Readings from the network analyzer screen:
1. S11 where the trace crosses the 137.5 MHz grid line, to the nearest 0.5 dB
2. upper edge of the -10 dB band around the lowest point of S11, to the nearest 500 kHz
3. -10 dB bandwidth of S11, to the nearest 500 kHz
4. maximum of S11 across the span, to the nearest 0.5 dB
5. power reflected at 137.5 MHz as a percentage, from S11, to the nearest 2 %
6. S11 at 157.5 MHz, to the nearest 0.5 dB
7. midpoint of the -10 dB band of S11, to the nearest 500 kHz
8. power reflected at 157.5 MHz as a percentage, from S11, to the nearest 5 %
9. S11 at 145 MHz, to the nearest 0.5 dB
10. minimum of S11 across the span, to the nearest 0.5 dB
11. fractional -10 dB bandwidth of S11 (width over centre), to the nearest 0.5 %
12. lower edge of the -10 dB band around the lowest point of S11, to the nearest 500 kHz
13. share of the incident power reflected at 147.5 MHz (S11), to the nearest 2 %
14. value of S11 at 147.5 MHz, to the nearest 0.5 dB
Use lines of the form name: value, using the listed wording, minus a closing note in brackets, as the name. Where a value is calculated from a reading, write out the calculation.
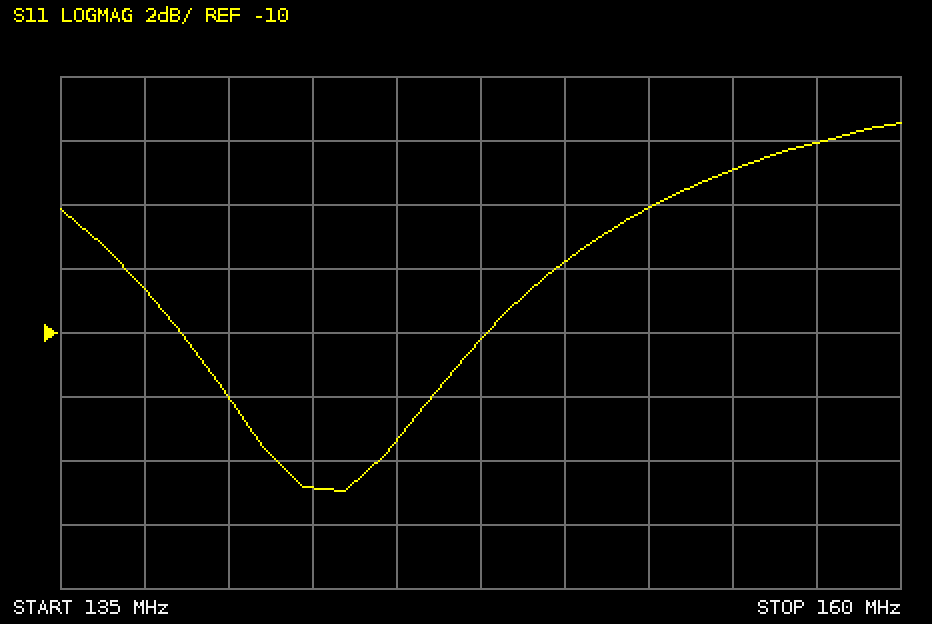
S11 where the trace crosses the 137.5 MHz grid line, to the nearest 0.5 dB: -8.5 dB
upper edge of the -10 dB band around the lowest point of S11, to the nearest 500 kHz: 147.5 MHz
-10 dB bandwidth of S11, to the nearest 500 kHz: 147.5 MHz − 138.5 MHz = 9.0 MHz
maximum of S11 across the span, to the nearest 0.5 dB: -3.5 dB
power reflected at 137.5 MHz as a percentage, from S11, to the nearest 2 %: 10^(-8.5/10) ≈ 14 %
S11 at 157.5 MHz, to the nearest 0.5 dB: -4.0 dB
midpoint of the -10 dB band of S11, to the nearest 500 kHz: 143.0 MHz
power reflected at 157.5 MHz as a percentage, from S11, to the nearest 5 %: 10^(-4/10) ≈ 40 %
S11 at 145 MHz, to the nearest 0.5 dB: -13.5 dB
minimum of S11 across the span, to the nearest 0.5 dB: -15.0 dB
fractional -10 dB bandwidth of S11 (width over centre), to the nearest 0.5 %: 9 MHz / 143 MHz ≈ 6.29 %, so 6.5 % to the nearest 0.5 %
lower edge of the -10 dB band around the lowest point of S11, to the nearest 500 kHz: 138.5 MHz
share of the incident power reflected at 147.5 MHz (S11), to the nearest 2 %: 10^(-10/10) ≈ 10 %
value of S11 at 147.5 MHz, to the nearest 0.5 dB: -10.0 dB
